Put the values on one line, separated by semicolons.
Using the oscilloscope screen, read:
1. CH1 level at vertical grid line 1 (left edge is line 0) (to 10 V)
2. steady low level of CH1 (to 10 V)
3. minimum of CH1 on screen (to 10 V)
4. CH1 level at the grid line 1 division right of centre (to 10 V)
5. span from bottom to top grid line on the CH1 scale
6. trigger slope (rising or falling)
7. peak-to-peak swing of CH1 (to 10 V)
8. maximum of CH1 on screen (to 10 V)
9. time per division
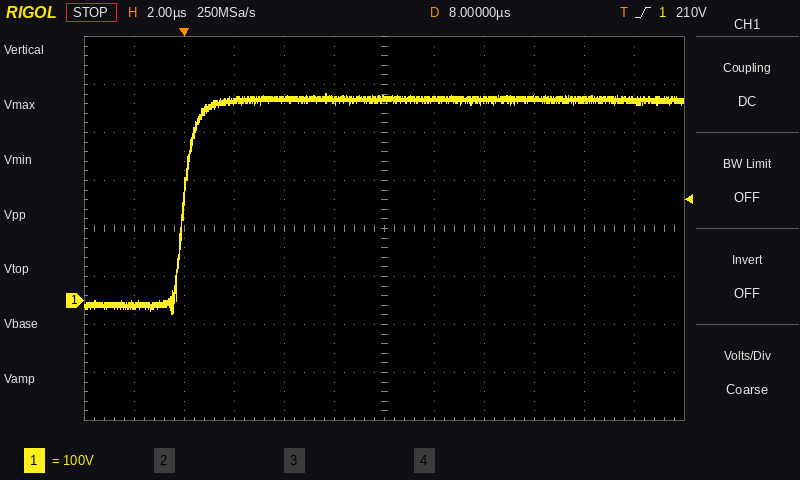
-10 V; -10 V; -30 V; 420 V; 800 V; rising; 460 V; 430 V; 2 µs
